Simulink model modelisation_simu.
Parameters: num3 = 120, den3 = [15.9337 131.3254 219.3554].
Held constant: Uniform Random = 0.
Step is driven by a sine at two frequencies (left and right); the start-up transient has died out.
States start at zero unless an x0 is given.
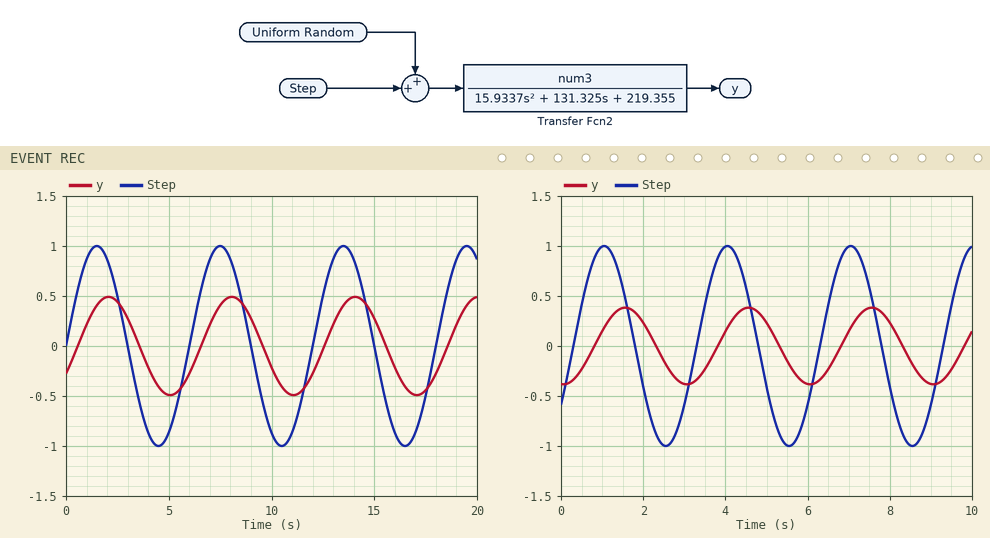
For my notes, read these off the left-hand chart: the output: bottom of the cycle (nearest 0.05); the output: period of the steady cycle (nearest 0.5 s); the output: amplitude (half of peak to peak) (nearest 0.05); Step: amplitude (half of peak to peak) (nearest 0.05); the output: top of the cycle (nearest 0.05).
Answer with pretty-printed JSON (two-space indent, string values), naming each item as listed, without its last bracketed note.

{
  "the output: bottom of the cycle": "-0.50",
  "the output: period of the steady cycle": "6.0 s",
  "the output: amplitude (half of peak to peak)": "0.50",
  "Step: amplitude (half of peak to peak)": "1.00",
  "the output: top of the cycle": "0.50"
}
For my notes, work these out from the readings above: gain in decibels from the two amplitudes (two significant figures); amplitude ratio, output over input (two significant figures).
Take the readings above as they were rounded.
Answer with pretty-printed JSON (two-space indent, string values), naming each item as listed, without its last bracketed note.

{
  "gain in decibels from the two amplitudes": "-6.0 dB",
  "amplitude ratio, output over input": "0.50"
}
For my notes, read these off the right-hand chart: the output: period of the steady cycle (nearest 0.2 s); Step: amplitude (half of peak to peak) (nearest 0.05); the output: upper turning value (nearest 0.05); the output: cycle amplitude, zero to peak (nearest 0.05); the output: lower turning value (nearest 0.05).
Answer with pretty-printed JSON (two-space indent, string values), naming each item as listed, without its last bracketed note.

{
  "the output: period of the steady cycle": "3.0 s",
  "Step: amplitude (half of peak to peak)": "1.00",
  "the output: upper turning value": "0.40",
  "the output: cycle amplitude, zero to peak": "0.40",
  "the output: lower turning value": "-0.40"
}
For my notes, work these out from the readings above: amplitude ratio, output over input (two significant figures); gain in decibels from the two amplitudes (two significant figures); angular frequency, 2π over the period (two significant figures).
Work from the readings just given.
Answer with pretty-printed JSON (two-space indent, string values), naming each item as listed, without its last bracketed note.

{
  "amplitude ratio, output over input": "0.40",
  "gain in decibels from the two amplitudes": "-8.0 dB",
  "angular frequency, 2π over the period": "2.1 rad/s"
}
